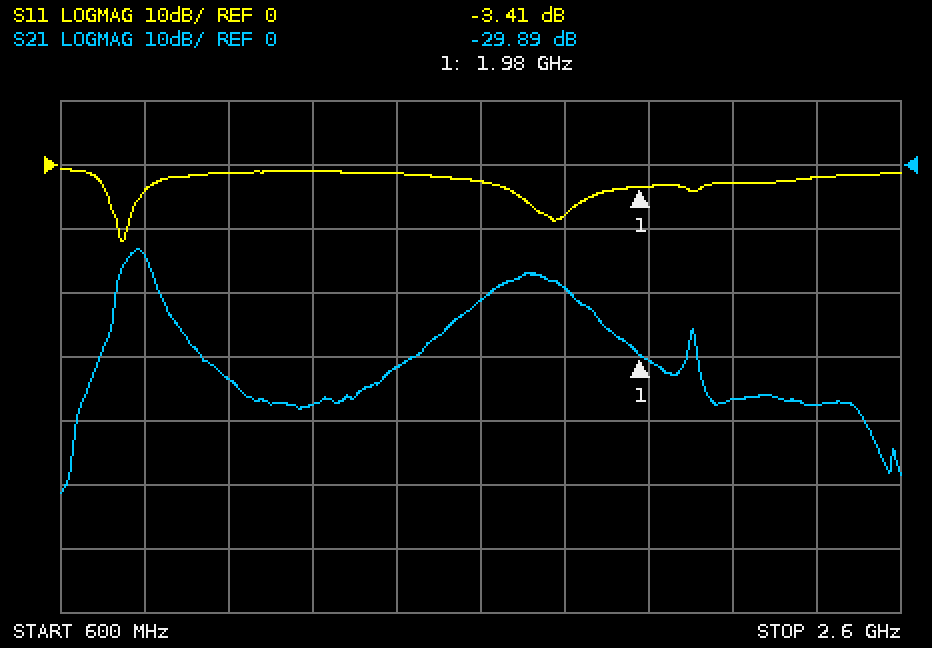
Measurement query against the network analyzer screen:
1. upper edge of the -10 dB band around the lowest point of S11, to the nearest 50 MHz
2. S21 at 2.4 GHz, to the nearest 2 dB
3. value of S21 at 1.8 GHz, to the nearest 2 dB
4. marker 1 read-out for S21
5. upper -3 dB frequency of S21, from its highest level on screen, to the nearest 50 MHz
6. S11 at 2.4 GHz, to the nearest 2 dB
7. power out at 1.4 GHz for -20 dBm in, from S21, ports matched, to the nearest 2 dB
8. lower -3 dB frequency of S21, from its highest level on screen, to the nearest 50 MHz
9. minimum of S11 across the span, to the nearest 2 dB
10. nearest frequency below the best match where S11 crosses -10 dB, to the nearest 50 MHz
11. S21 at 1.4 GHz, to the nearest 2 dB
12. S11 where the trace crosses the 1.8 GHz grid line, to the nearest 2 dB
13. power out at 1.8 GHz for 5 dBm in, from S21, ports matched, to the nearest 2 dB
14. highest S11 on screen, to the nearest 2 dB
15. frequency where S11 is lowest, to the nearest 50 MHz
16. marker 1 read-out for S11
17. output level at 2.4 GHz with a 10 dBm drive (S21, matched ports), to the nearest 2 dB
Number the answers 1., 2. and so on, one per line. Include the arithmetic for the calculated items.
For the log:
1. 750 MHz
2. -38 dB
3. -20 dB
4. -29.89 dB
5. 800 MHz
6. -2 dB
7. -20 dBm + (-32 dB) = -52 dBm
8. 750 MHz
9. -12 dB
10. 750 MHz
11. -32 dB
12. -8 dB
13. 5 dBm + (-20 dB) = -14 dBm
14. 0 dB
15. 750 MHz
16. -3.41 dB
17. 10 dBm + (-38 dB) = -28 dBm
